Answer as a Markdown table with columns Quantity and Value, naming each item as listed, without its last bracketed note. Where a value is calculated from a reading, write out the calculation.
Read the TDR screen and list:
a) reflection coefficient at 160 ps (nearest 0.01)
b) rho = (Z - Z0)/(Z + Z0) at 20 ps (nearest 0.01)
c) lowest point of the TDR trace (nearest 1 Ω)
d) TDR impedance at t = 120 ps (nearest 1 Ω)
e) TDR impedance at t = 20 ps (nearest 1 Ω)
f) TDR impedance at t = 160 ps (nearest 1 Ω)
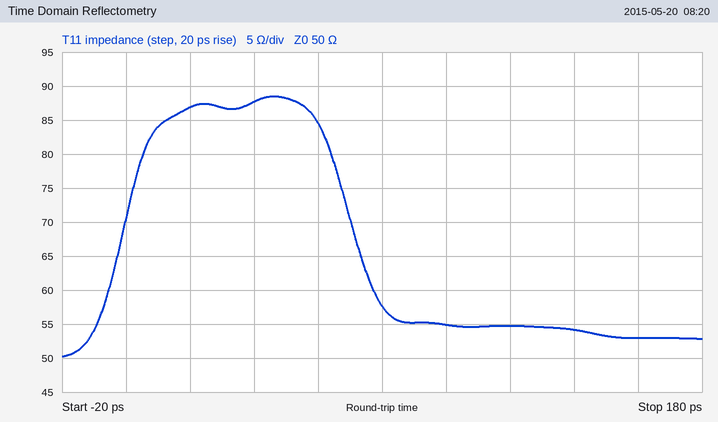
| Quantity | Value |
|---|---|
| reflection coefficient at 160 ps | (53 − 50)/(53 + 50) ≈ +0.03 |
| rho = (Z - Z0)/(Z + Z0) at 20 ps | (87 − 50)/(87 + 50) ≈ +0.27 |
| lowest point of the TDR trace | 50 Ω |
| TDR impedance at t = 120 ps | 55 Ω |
| TDR impedance at t = 20 ps | 87 Ω |
| TDR impedance at t = 160 ps | 53 Ω |
